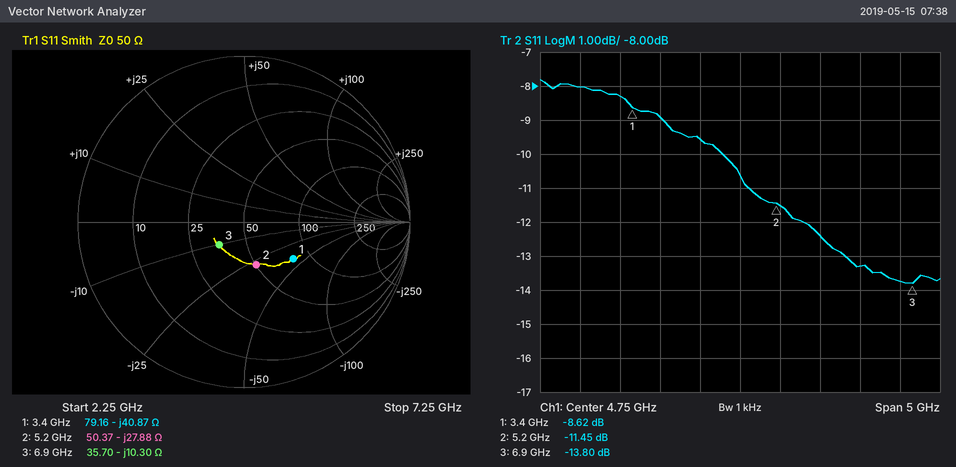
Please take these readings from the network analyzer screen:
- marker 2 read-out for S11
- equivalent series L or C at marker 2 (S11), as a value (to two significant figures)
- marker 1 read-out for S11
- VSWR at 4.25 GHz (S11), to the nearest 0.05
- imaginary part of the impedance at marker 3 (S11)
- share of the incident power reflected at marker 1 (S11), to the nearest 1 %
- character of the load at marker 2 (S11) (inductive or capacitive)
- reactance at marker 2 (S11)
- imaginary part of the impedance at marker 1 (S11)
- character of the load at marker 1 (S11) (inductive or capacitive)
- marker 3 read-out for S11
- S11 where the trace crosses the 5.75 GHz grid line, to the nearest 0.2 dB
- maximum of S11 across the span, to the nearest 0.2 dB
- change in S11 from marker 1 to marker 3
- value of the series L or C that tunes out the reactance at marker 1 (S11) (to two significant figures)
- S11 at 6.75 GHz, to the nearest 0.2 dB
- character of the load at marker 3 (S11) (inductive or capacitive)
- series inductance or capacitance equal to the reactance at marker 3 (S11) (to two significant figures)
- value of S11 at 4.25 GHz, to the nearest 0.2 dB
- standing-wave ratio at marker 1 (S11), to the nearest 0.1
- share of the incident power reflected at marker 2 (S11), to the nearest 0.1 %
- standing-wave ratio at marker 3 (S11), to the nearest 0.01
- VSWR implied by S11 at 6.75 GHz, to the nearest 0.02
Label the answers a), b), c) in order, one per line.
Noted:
a) -11.45 dB
b) 1.1 pF
c) -8.62 dB
d) 2.00
e) -10.30 Ω
f) 14 %
g) capacitive
h) -27.88 Ω
i) -40.87 Ω
j) capacitive
k) -13.80 dB
l) -12.4 dB
m) -7.8 dB
n) -5.18 dB
o) 1.9 nH
p) -13.8 dB
q) capacitive
r) 2.2 pF
s) -9.6 dB
t) 2.2
u) 7.2 %
v) 1.51
w) 1.52
